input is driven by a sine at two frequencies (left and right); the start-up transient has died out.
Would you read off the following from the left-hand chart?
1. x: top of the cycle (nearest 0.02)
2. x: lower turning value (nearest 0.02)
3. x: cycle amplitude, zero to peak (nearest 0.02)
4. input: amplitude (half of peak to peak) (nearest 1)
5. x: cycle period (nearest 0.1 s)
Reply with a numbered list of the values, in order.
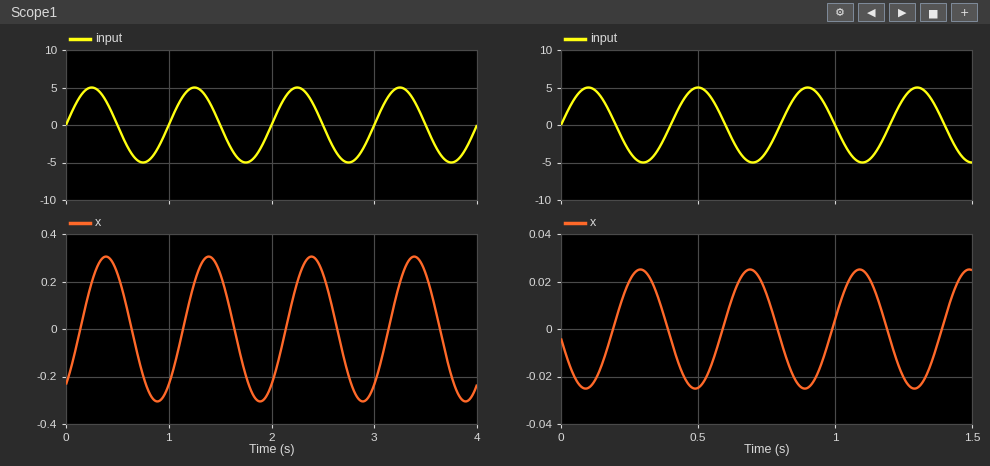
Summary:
1. 0.30
2. -0.30
3. 0.30
4. 5
5. 1.0 s
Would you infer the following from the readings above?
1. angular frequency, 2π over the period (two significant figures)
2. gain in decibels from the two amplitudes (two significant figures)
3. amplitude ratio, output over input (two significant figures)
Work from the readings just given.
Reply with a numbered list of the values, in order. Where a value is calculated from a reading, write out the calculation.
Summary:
1. 2π / 1 = 6.3 rad/s
2. 20 log10(0.3 / 5) = -24 dB
3. 0.3 / 5 = 0.060
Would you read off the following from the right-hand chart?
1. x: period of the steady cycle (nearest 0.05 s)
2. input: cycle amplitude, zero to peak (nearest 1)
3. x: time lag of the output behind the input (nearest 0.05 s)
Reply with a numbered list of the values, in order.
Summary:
1. 0.40 s
2. 5
3. 0.20 s
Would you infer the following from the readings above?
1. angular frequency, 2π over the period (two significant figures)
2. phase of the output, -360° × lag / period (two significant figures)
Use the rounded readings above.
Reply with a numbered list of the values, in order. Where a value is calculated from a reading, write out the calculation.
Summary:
1. 2π / 0.4 = 16 rad/s
2. -360 × 0.2 / 0.4 = -180°
